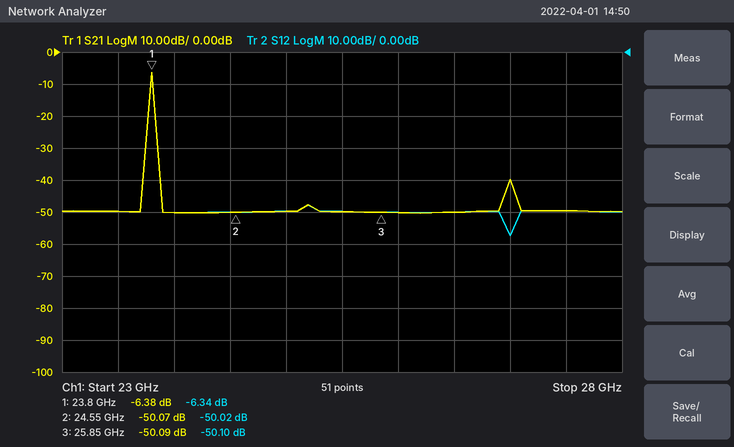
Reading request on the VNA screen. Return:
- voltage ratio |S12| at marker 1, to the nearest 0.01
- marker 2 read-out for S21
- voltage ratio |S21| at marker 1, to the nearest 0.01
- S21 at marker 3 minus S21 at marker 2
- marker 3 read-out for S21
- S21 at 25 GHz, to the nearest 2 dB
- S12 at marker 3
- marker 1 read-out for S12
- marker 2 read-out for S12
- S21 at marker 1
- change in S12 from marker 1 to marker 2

0.48
-50.07 dB
0.48
-0.02 dB
-50.09 dB
-50 dB
-50.10 dB
-6.34 dB
-50.02 dB
-6.38 dB
-43.68 dB
